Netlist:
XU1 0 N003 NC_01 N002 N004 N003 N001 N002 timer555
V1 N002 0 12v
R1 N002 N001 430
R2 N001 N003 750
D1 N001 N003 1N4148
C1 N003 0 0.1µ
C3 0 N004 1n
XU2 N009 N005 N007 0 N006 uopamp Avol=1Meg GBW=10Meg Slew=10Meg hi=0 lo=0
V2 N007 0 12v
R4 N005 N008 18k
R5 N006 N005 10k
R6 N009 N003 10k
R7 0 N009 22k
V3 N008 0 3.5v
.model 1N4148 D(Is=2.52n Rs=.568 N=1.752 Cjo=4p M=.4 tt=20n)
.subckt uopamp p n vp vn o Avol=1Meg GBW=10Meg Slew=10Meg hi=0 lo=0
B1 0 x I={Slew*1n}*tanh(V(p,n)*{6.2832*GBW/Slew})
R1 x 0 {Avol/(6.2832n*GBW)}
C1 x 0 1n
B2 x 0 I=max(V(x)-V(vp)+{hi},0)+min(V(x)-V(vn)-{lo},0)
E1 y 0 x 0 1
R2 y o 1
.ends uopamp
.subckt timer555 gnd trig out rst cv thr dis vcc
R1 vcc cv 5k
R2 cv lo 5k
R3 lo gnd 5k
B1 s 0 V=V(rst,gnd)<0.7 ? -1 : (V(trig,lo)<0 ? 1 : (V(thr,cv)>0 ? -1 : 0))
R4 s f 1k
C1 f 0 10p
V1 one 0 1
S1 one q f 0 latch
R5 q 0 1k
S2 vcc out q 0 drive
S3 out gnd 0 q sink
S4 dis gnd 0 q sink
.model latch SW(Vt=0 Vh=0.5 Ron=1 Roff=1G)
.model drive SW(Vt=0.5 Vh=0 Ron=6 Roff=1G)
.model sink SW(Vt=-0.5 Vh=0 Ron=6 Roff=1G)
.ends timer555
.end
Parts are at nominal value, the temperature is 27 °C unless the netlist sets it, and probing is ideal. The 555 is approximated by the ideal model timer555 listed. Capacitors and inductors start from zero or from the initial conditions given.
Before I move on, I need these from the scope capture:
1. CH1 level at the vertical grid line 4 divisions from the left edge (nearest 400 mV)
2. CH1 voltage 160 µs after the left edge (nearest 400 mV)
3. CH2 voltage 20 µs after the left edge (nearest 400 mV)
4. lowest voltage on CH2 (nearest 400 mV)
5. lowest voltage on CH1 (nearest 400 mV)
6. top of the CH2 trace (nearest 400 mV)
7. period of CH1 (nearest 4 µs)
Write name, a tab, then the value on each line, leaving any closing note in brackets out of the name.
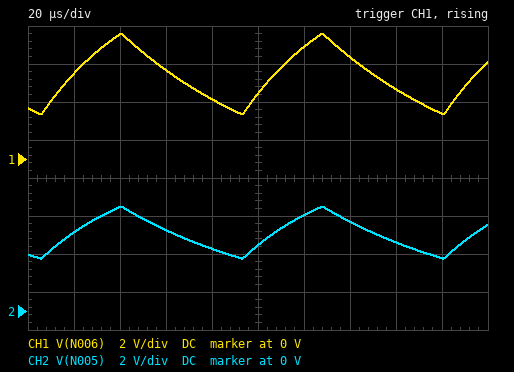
CH1 level at the vertical grid line 4 divisions from the left edge	3.2 V
CH1 voltage 160 µs after the left edge	3.6 V
CH2 voltage 20 µs after the left edge	4.0 V
lowest voltage on CH2	2.8 V
lowest voltage on CH1	2.4 V
top of the CH2 trace	5.6 V
period of CH1	88 µs
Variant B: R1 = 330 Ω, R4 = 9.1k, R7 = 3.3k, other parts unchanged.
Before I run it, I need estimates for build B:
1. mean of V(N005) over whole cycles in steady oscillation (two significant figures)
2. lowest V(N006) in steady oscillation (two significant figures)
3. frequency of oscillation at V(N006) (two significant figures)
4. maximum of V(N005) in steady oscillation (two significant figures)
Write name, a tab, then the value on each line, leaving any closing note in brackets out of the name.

mean of V(N005) over whole cycles in steady oscillation	1.8 V
lowest V(N006) in steady oscillation	-9.8 mV
frequency of oscillation at V(N006)	13 kHz
maximum of V(N005) in steady oscillation	2.0 V
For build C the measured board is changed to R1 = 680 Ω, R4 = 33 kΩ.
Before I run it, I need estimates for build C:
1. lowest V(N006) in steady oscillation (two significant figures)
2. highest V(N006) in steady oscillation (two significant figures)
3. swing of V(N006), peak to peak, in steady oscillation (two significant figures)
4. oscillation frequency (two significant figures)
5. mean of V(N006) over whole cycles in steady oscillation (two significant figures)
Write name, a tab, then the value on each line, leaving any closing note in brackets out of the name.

lowest V(N006) in steady oscillation	2.5 V
highest V(N006) in steady oscillation	6.1 V
swing of V(N006), peak to peak, in steady oscillation	3.6 V
oscillation frequency	9.3 kHz
mean of V(N006) over whole cycles in steady oscillation	4.3 V
